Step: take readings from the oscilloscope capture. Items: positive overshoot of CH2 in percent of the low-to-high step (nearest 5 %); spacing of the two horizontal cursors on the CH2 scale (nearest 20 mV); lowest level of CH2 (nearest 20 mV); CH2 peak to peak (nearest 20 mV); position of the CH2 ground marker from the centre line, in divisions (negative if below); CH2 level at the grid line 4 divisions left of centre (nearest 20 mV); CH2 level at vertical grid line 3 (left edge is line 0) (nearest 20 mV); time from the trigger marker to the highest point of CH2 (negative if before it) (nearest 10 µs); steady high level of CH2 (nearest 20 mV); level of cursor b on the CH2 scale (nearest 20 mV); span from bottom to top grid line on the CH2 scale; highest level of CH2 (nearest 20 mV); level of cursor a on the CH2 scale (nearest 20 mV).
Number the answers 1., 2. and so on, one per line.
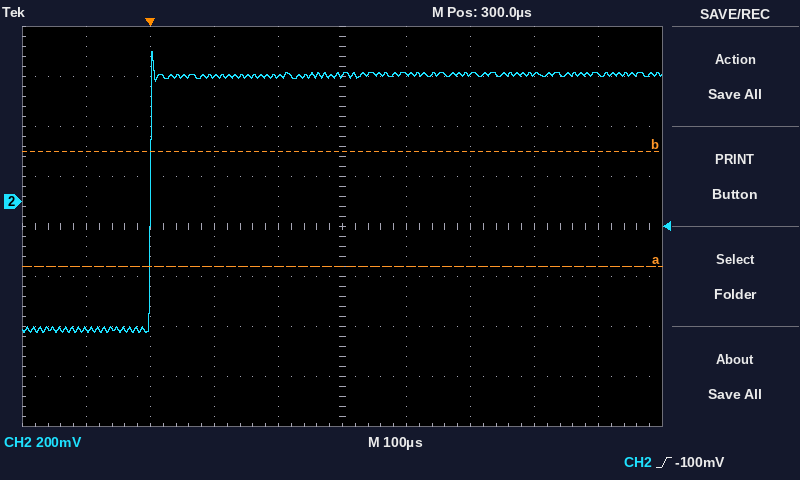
1. 10 %
2. 460 mV
3. -520 mV
4. 1.12 V
5. +0.5 div
6. -520 mV
7. 500 mV
8. 0 µs
9. 500 mV
10. 200 mV
11. 1.6 V
12. 600 mV
13. -260 mV
